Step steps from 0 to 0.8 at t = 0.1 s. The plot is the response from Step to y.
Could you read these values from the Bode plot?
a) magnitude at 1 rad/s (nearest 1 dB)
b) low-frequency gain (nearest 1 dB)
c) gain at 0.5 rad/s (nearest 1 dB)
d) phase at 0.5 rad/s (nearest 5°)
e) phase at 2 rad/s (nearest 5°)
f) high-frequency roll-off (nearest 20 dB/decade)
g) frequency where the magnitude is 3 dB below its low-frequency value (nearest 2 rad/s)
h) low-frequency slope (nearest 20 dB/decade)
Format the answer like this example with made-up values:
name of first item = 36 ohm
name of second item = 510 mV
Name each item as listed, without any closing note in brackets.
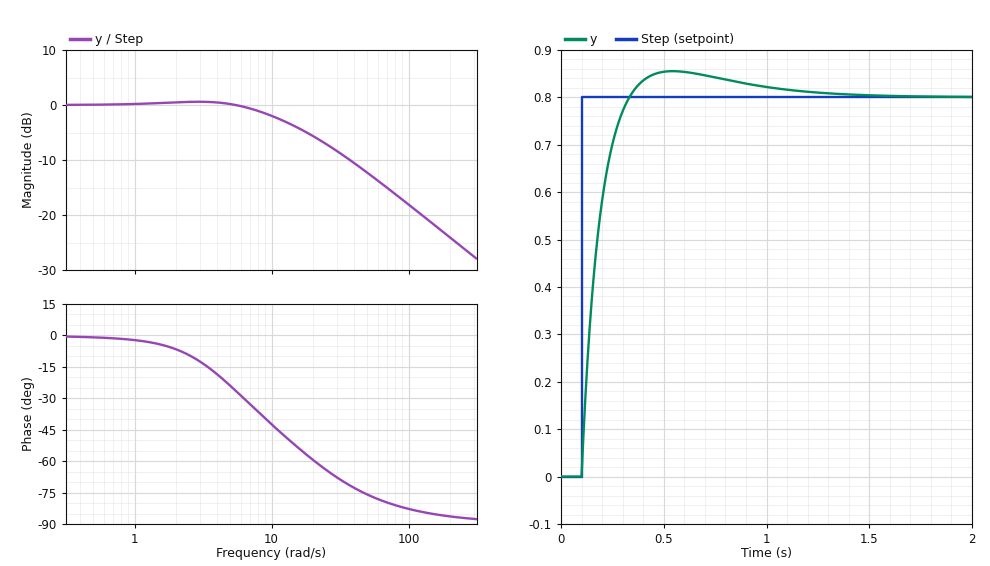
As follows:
magnitude at 1 rad/s = 0 dB
low-frequency gain = 0 dB
gain at 0.5 rad/s = 0 dB
phase at 0.5 rad/s = 0°
phase at 2 rad/s = -5°
high-frequency roll-off = -20 dB/decade
frequency where the magnitude is 3 dB below its low-frequency value = 12 rad/s
low-frequency slope = 0 dB/decade
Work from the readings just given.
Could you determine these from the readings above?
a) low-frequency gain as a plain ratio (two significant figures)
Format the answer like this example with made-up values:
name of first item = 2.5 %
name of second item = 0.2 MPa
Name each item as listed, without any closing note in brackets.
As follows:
low-frequency gain as a plain ratio = 1.0
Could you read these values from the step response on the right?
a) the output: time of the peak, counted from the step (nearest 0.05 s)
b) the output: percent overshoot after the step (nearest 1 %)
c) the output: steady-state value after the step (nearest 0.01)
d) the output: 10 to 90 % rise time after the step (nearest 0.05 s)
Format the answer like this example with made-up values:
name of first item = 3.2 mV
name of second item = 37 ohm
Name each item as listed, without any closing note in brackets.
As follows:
the output: time of the peak, counted from the step = 0.45 s
the output: percent overshoot after the step = 7 %
the output: steady-state value after the step = 0.80
the output: 10 to 90 % rise time after the step = 0.15 s
